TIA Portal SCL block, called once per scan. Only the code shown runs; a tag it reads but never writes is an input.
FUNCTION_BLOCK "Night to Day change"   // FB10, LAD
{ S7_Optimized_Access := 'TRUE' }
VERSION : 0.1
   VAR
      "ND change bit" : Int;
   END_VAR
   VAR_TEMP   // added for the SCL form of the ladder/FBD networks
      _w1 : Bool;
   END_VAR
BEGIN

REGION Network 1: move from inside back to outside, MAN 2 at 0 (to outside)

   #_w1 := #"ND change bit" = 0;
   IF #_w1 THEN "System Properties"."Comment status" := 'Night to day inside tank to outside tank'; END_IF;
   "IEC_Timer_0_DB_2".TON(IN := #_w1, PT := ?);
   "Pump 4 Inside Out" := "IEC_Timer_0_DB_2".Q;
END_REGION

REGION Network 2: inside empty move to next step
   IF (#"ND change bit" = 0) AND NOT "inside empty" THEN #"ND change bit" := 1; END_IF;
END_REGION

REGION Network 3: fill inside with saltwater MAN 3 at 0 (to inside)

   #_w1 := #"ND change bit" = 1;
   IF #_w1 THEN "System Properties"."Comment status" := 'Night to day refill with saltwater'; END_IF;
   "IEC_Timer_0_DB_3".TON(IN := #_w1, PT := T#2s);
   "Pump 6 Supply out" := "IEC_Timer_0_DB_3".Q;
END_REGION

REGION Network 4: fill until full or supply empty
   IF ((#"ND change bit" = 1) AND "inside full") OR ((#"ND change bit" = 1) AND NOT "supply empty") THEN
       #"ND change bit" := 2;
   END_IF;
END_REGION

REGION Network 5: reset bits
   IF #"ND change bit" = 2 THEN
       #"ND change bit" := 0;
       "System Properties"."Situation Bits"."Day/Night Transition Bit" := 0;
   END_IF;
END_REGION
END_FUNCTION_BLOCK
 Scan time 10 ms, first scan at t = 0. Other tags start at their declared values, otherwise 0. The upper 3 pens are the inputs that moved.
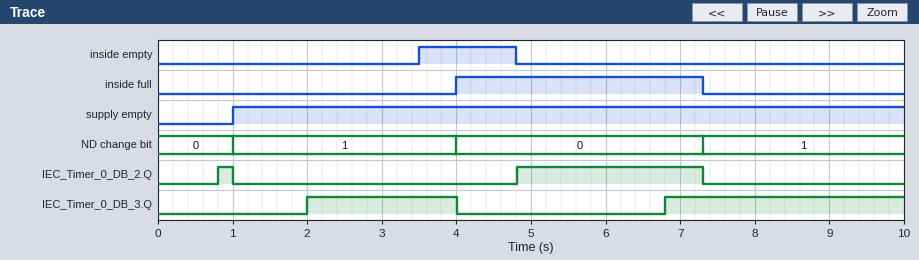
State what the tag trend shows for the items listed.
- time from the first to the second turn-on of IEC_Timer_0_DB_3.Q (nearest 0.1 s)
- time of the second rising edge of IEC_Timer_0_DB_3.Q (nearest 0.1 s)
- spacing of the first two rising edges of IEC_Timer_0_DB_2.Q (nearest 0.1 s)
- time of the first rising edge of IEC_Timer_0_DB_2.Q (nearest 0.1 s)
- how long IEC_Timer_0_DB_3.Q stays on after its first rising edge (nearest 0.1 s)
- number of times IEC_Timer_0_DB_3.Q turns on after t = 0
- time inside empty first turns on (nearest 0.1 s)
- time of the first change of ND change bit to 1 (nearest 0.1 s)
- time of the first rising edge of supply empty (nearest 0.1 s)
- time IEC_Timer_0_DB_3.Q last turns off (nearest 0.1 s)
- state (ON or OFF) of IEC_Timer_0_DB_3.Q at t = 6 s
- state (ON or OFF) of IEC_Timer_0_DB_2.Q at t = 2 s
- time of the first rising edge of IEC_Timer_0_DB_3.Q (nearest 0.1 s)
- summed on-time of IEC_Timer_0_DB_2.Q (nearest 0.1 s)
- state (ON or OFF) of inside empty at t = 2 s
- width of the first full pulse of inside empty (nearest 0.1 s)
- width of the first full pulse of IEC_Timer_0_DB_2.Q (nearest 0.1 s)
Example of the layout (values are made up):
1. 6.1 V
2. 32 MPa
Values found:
1. 4.8 s
2. 6.8 s
3. 4.0 s
4. 0.8 s
5. 2.0 s
6. 2
7. 3.5 s
8. 1.0 s
9. 1.0 s
10. 4.0 s
11. OFF
12. OFF
13. 2.0 s
14. 2.7 s
15. OFF
16. 1.3 s
17. 0.2 s
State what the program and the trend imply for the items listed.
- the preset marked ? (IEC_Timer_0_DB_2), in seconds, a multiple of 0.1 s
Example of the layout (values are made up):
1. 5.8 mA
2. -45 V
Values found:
1. 0.8 s
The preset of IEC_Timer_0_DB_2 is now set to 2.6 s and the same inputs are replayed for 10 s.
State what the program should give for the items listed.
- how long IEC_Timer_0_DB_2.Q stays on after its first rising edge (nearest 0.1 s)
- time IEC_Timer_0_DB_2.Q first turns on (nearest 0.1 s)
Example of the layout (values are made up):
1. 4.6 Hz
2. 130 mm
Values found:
1. 0.7 s
2. 6.6 s
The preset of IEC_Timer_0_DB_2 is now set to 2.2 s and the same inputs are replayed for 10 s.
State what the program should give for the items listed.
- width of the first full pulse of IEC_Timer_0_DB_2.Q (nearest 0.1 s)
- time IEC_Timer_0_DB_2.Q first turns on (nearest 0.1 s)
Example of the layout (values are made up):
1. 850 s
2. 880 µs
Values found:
1. 1.1 s
2. 6.2 s
